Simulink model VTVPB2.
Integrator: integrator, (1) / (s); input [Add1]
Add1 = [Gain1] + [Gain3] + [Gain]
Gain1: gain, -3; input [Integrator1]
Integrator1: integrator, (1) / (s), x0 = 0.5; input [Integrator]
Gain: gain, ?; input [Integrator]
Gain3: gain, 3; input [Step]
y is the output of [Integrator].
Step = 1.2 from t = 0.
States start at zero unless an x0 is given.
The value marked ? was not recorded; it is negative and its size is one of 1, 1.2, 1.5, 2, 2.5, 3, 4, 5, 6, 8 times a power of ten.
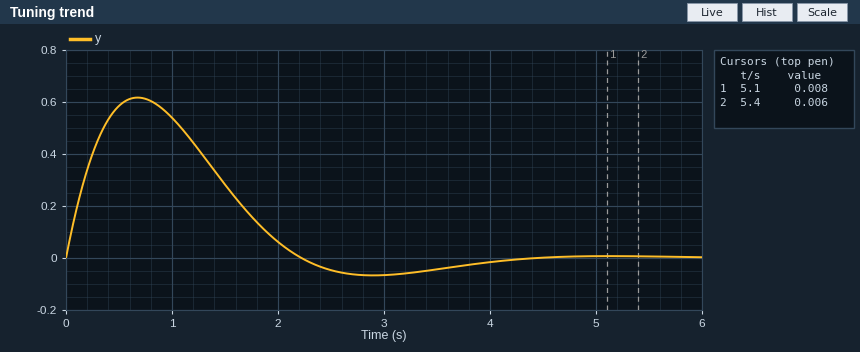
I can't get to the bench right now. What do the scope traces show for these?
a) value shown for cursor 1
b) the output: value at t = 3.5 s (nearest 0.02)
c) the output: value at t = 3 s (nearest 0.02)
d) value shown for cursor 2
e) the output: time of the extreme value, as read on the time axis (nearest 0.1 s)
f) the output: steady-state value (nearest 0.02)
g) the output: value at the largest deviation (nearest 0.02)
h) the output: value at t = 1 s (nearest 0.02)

0.008
-0.04
-0.06
0.006
0.7 s
0.00
0.62
0.54
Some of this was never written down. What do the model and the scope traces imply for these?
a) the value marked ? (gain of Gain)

-2
